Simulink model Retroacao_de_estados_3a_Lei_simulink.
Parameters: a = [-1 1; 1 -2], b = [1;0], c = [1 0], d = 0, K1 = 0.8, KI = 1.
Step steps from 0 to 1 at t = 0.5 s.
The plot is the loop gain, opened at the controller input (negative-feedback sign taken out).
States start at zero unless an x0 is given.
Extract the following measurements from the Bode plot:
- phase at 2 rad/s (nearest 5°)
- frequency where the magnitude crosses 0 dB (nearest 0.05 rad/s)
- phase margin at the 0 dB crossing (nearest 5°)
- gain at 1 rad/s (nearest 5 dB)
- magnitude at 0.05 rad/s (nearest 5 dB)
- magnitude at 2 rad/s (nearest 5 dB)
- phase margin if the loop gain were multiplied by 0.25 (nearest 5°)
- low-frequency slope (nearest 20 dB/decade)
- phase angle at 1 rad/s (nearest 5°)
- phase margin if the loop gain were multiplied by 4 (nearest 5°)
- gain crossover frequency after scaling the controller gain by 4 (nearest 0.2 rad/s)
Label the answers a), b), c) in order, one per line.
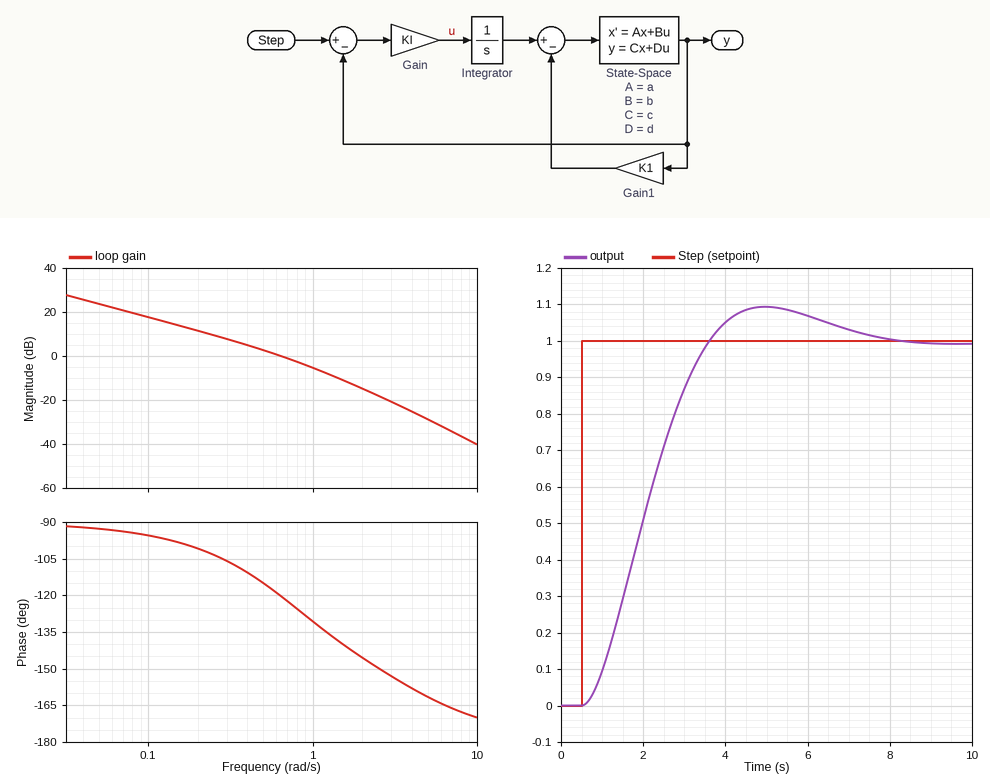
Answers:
a) -145°
b) 0.65 rad/s
c) 60°
d) -5 dB
e) 25 dB
f) -15 dB
g) 80°
h) -20 dB/decade
i) -130°
j) 40°
k) 1.6 rad/s
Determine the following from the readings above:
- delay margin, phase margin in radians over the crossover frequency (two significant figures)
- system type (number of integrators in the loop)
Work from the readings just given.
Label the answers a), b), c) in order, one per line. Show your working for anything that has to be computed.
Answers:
a) 60 × π / 180 / 0.65 = 1.6 s
b) 1
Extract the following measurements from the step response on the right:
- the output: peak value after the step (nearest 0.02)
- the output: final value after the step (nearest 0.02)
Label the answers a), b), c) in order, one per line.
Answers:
a) 1.10
b) 1.00
